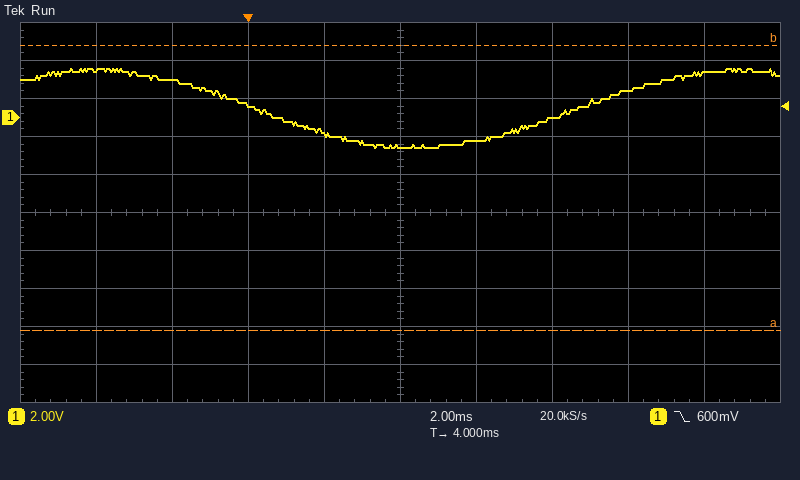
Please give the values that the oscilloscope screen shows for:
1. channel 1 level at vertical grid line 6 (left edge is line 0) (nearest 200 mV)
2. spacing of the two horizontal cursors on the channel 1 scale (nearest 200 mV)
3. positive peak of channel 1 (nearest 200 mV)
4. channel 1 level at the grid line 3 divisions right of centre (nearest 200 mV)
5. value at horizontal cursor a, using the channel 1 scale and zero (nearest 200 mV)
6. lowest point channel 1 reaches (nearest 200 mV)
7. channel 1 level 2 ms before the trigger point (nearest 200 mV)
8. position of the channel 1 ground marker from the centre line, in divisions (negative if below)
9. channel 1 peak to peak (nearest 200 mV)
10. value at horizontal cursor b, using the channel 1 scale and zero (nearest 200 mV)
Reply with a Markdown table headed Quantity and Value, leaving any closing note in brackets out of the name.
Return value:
| Quantity | Value |
|---|---|
| channel 1 level at vertical grid line 6 (left edge is line 0) | -1.2 V |
| spacing of the two horizontal cursors on the channel 1 scale | 15.0 V |
| positive peak of channel 1 | 2.6 V |
| channel 1 level at the grid line 3 divisions right of centre | 1.4 V |
| value at horizontal cursor a, using the channel 1 scale and zero | -11.2 V |
| lowest point channel 1 reaches | -1.6 V |
| channel 1 level 2 ms before the trigger point | 2.0 V |
| position of the channel 1 ground marker from the centre line, in divisions | +2.5 div |
| channel 1 peak to peak | 4.2 V |
| value at horizontal cursor b, using the channel 1 scale and zero | 3.8 V |
